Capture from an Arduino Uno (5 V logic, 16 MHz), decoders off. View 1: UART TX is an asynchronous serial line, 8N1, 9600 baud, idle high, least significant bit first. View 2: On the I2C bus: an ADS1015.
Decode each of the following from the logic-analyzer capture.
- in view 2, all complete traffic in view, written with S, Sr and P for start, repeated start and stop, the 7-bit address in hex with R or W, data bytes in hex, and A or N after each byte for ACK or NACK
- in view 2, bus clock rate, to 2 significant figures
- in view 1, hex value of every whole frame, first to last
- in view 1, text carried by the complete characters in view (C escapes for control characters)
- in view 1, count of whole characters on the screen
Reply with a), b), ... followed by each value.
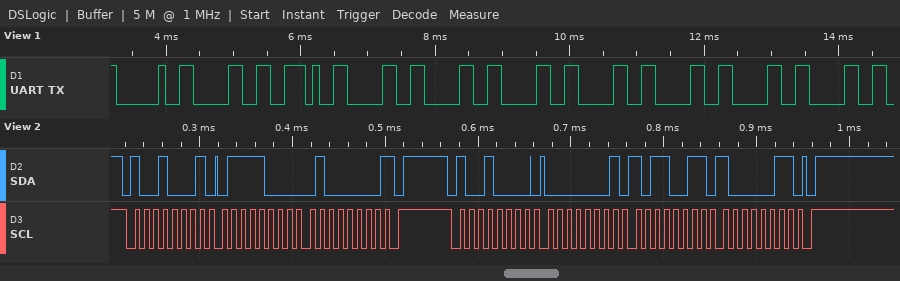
a) S 48R A 78 A 40 N P S 48W A 01 A B3 A 83 A P
b) 100 kHz
c) 20 30 2E 30 30 30 30 30 30 30
d) " 0.0000000"
e) 10
